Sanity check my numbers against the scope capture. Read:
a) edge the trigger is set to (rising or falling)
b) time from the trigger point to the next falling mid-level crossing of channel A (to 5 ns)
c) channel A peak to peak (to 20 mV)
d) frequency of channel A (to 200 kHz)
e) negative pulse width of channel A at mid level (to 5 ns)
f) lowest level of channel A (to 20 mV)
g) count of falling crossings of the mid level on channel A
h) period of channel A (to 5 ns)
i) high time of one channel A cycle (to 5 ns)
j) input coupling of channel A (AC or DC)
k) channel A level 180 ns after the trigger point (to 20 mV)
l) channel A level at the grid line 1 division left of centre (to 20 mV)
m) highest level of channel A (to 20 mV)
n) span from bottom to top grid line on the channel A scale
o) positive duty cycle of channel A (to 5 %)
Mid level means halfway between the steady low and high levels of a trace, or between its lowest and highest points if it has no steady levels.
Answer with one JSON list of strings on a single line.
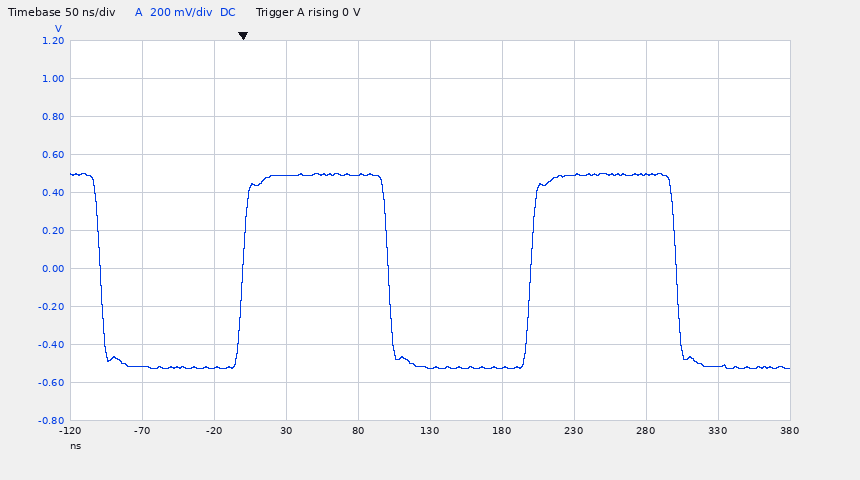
["rising", "100 ns", "1.02 V", "5.0 MHz", "100 ns", "-520 mV", "3", "200 ns", "100 ns", "DC", "-520 mV", "500 mV", "500 mV", "2 V", "50 %"]
